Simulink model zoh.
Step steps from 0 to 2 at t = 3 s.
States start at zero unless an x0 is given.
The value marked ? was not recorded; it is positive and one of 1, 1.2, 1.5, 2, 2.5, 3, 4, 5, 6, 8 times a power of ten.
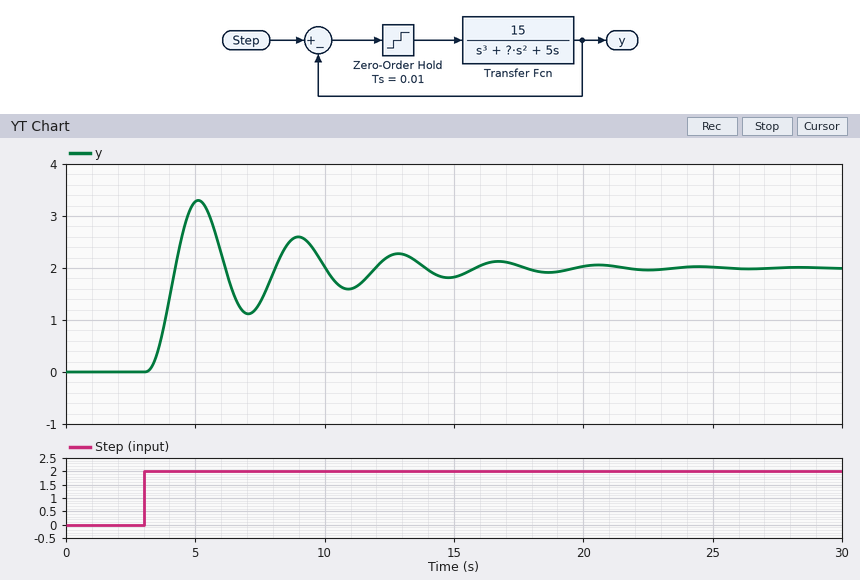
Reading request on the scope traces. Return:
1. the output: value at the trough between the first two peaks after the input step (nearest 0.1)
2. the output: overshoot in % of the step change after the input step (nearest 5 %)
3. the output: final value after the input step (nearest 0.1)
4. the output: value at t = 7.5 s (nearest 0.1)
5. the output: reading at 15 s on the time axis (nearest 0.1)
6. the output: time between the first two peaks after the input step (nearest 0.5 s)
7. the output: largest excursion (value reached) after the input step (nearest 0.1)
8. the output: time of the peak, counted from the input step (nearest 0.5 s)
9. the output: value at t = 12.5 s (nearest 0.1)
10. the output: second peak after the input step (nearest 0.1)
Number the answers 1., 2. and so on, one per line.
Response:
1. 1.1
2. 65 %
3. 2.0
4. 1.3
5. 1.8
6. 4.0 s
7. 3.3
8. 2.0 s
9. 2.2
10. 2.6
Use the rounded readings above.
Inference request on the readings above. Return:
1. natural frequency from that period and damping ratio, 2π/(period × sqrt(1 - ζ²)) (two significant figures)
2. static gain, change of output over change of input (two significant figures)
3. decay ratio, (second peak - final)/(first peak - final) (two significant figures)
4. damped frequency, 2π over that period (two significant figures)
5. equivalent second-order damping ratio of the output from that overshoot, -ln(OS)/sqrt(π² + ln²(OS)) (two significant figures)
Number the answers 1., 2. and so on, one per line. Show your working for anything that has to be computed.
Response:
1. 2π / (4 × sqrt(1 - 0.14²)) = 1.6 rad/s
2. (2 - 0) / (2 - 0) = 1.0
3. (2.6 - 2) / (3.3 - 2) = 0.46
4. 2π / 4 = 1.6 rad/s
5. ln(0.65) = -0.431; 0.431 / sqrt(9.870 + 0.186) = 0.14
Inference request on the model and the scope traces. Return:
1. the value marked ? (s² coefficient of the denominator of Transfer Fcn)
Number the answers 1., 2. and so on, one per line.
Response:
1. 6
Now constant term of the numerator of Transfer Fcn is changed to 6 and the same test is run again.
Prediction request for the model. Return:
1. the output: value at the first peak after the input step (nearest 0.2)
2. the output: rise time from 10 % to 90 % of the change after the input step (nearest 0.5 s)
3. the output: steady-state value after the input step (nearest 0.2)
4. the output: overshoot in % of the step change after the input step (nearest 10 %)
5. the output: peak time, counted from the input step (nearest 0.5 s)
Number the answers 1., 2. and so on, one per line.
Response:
1. 2.6
2. 1.5 s
3. 2.0
4. 30 %
5. 3.5 s
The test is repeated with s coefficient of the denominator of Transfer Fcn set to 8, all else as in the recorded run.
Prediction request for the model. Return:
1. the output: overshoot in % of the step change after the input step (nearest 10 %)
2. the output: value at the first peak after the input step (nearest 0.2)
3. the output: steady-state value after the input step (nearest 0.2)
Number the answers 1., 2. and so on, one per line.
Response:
1. 40 %
2. 2.8
3. 2.0
